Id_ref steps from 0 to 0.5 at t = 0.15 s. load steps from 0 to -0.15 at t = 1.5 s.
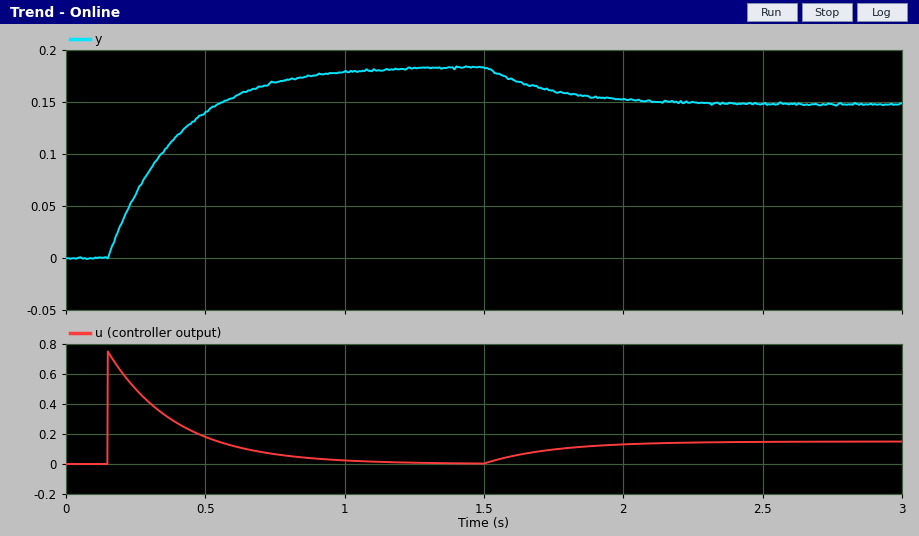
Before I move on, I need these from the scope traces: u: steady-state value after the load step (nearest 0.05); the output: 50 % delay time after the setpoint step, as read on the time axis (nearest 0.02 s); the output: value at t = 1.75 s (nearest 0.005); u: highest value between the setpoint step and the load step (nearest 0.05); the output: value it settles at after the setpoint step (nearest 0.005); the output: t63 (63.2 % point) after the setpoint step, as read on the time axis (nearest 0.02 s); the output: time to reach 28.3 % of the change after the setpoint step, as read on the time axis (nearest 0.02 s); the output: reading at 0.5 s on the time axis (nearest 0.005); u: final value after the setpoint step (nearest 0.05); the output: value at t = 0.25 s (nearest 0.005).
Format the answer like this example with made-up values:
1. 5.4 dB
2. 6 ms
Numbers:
1. 0.15
2. 0.32 s
3. 0.160
4. 0.75
5. 0.185
6. 0.40 s
7. 0.24 s
8. 0.140
9. 0.00
10. 0.060
